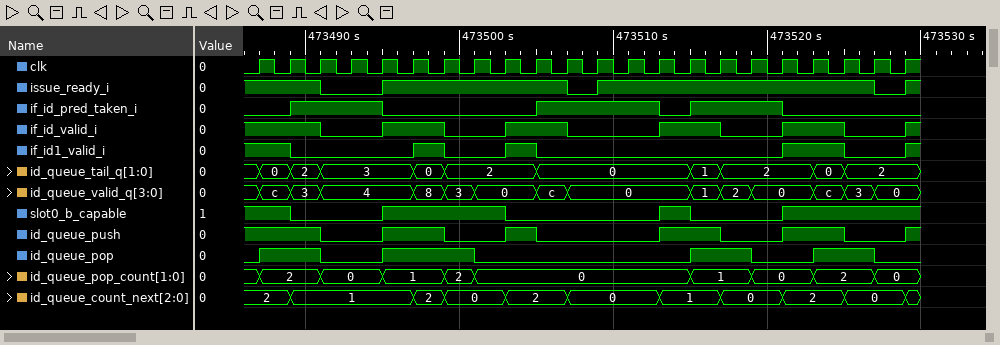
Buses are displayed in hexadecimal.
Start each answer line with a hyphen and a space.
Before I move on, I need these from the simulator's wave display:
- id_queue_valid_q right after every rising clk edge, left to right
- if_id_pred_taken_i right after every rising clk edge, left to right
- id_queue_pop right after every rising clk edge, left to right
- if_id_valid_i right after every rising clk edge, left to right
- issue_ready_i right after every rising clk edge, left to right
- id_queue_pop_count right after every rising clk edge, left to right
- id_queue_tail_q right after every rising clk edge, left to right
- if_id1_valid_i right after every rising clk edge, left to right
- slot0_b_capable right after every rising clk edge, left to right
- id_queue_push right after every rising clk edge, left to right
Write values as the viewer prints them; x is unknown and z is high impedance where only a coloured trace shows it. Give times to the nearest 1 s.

- c, 3, 4, 4, 4, 8, 3, 0, 0, c, 0, 0, 0, 0, 1, 2, 0, 0, c, 3, 0, 0
- 0 1 1 1 0 0 0 0 0 1 1 1 1 0 1 1 1 0 0 0 0 0
- 1 1 0 0 1 1 1 0 0 0 0 0 0 0 1 1 0 0 1 1 0 0
- 1 1 0 0 1 1 0 0 1 1 0 0 0 1 1 0 0 1 1 0 0 1
- 1 1 0 0 1 1 1 1 1 1 0 1 1 1 1 1 1 1 1 1 0 1
- 2, 2, 0, 0, 1, 1, 2, 0, 0, 0, 0, 0, 0, 0, 1, 1, 0, 0, 2, 2, 0, 0
- 0, 2, 3, 3, 3, 0, 2, 2, 2, 0, 0, 0, 0, 0, 1, 2, 2, 2, 0, 2, 2, 2
- 1 0 0 0 0 1 0 0 1 0 0 0 0 0 0 0 0 1 1 0 0 1
- 1 0 0 0 1 1 1 1 0 0 0 0 0 1 0 0 0 1 1 1 1 1
- 1 1 0 0 1 1 0 0 1 0 0 0 0 1 1 0 0 1 1 0 0 1
